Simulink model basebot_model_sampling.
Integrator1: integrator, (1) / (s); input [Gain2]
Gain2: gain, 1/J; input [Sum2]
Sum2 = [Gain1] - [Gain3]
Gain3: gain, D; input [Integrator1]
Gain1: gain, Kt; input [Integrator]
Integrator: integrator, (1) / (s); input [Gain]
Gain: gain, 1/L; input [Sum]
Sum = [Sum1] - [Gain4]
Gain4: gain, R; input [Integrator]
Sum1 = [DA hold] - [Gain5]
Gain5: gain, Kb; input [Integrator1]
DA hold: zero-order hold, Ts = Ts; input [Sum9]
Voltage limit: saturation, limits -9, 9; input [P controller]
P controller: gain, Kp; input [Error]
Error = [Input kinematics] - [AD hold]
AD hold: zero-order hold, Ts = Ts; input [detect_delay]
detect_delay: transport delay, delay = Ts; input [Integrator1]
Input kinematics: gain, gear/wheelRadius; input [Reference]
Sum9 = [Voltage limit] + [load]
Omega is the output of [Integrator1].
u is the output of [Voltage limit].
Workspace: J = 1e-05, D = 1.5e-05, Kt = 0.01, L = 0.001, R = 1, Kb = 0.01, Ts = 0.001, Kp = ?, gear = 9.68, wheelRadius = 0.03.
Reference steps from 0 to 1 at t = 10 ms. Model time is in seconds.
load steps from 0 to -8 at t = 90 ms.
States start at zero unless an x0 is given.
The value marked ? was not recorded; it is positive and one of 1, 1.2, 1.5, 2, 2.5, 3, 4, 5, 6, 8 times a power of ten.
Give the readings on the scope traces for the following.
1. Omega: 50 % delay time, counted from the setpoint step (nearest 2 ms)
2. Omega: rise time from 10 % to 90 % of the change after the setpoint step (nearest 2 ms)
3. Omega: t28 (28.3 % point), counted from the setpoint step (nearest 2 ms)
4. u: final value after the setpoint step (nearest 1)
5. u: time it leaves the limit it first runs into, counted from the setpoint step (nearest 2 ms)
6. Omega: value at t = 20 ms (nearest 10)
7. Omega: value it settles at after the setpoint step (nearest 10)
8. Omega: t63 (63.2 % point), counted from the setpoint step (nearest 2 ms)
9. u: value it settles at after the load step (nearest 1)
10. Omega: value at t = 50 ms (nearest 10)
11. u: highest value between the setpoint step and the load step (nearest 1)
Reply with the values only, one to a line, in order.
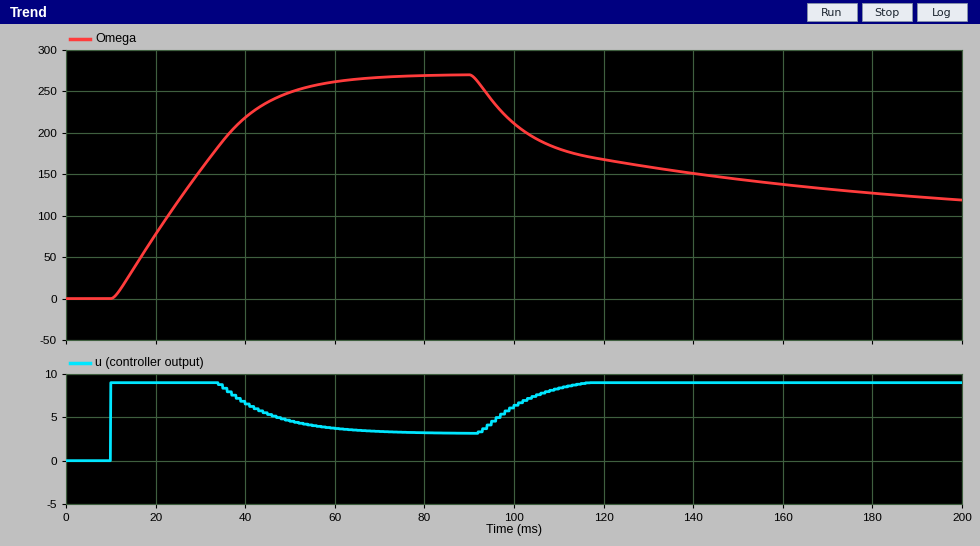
18 ms
34 ms
10 ms
3
24 ms
80
270
22 ms
9
250
9
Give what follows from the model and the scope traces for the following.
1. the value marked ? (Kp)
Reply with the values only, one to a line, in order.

0.06
